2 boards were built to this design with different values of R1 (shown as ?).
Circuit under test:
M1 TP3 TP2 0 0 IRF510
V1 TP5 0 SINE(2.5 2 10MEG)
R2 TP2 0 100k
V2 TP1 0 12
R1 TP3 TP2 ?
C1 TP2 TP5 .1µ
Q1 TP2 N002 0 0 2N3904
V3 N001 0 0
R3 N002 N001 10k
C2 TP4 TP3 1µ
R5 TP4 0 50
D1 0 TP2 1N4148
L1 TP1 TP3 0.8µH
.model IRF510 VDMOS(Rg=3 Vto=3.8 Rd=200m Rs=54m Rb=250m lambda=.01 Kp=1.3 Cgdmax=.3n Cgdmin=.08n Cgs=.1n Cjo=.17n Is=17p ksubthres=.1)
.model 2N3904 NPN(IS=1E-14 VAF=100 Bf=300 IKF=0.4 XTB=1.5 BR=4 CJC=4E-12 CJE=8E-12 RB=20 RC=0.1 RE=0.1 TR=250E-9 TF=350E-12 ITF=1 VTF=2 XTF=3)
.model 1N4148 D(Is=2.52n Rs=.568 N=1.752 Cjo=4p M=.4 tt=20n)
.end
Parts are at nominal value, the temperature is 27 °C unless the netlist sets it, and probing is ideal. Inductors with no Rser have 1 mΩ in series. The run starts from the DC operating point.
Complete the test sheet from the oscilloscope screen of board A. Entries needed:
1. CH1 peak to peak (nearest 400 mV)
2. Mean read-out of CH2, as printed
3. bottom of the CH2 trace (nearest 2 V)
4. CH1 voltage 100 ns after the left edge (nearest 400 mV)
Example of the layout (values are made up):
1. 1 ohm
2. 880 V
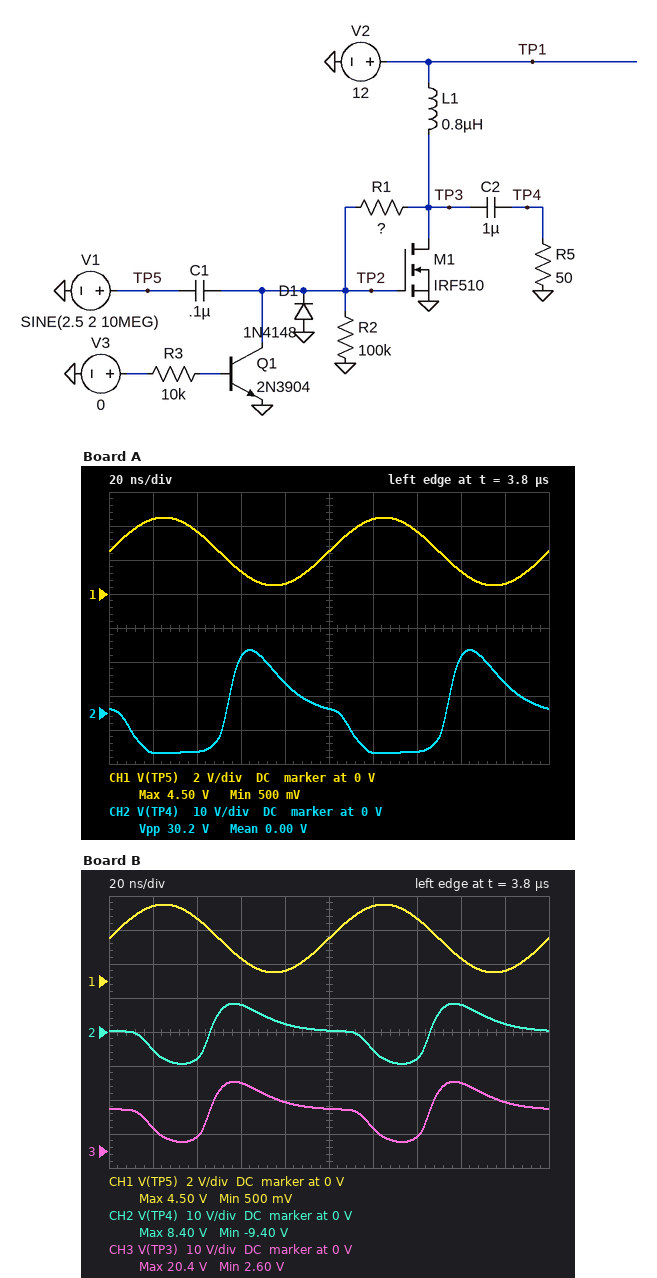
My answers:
1. 4.0 V
2. 0.00 V
3. -12 V
4. 2.4 V
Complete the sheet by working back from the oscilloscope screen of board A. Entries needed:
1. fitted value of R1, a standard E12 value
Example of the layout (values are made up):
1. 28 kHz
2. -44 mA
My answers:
1. 220 kΩ
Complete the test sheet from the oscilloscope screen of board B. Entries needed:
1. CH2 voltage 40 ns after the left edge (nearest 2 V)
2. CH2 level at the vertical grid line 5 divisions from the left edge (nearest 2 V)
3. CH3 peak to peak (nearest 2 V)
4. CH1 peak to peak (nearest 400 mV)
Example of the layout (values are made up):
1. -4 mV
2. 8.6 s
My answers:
1. -8 V
2. 0 V
3. 18 V
4. 4.0 V
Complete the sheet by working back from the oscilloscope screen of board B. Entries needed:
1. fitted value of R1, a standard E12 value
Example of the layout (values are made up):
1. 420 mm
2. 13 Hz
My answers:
1. 330 kΩ
